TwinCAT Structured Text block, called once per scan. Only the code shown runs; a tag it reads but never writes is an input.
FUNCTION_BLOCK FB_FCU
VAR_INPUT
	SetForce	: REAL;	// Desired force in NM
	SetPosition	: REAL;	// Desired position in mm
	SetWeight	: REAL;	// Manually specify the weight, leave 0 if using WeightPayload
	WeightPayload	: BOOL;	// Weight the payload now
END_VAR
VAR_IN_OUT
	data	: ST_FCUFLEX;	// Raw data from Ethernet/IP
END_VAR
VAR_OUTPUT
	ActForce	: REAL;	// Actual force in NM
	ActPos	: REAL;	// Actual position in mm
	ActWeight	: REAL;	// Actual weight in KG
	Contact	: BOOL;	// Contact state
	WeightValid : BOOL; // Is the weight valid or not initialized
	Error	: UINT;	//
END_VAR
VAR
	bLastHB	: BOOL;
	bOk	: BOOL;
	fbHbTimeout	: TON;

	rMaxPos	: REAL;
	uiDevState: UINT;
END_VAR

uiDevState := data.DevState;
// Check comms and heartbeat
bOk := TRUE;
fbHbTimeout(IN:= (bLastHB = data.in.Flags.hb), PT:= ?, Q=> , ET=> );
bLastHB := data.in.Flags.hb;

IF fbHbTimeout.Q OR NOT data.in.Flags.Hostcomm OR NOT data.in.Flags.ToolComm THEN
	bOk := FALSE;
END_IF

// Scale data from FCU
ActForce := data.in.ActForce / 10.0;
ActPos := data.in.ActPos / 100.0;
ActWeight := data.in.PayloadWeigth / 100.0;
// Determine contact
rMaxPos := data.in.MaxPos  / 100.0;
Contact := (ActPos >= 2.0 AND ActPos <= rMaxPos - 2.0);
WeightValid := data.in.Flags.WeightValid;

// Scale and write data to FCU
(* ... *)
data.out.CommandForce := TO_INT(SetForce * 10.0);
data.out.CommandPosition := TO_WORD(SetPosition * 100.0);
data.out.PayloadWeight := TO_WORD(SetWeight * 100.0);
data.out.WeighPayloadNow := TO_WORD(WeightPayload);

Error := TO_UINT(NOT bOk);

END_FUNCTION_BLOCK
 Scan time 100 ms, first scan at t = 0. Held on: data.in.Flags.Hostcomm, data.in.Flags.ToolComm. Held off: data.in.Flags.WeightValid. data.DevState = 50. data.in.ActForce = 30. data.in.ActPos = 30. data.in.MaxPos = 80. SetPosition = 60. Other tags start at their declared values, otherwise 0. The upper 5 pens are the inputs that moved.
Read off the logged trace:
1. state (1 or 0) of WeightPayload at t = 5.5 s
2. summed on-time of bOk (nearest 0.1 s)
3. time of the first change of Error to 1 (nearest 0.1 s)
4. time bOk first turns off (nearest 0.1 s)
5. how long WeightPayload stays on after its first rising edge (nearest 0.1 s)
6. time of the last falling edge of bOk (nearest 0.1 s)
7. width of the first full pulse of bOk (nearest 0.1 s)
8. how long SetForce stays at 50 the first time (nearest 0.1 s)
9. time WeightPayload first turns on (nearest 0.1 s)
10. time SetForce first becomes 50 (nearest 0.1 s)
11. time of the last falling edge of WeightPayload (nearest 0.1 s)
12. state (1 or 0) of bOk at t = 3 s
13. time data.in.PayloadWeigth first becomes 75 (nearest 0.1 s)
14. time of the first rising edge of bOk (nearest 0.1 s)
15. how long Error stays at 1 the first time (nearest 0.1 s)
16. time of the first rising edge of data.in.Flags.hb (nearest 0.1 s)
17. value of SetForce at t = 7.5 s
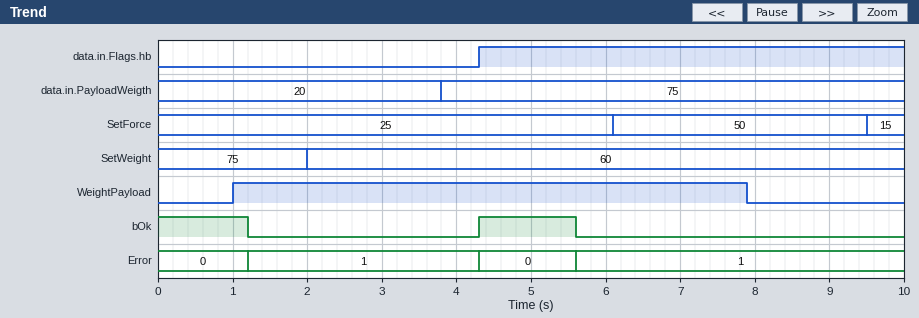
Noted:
1
2.5 s
1.2 s
1.2 s
6.9 s
5.6 s
1.3 s
3.4 s
1.0 s
6.1 s
7.9 s
0
3.8 s
4.3 s
3.1 s
4.3 s
50
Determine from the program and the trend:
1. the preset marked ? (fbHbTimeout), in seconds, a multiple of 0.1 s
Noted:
1.2 s
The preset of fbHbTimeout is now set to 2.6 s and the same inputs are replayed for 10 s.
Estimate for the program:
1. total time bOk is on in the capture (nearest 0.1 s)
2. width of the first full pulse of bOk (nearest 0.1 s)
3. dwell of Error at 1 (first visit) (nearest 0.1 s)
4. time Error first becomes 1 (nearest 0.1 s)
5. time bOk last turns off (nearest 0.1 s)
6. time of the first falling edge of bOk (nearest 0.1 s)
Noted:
5.3 s
2.7 s
1.7 s
2.6 s
7.0 s
2.6 s
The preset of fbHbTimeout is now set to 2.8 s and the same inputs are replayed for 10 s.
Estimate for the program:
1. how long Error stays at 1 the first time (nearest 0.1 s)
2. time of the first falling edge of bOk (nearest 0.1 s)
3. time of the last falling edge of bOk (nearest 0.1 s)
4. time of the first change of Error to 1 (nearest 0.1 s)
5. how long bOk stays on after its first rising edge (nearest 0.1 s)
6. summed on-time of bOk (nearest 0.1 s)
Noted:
1.5 s
2.8 s
7.2 s
2.8 s
2.9 s
5.7 s
